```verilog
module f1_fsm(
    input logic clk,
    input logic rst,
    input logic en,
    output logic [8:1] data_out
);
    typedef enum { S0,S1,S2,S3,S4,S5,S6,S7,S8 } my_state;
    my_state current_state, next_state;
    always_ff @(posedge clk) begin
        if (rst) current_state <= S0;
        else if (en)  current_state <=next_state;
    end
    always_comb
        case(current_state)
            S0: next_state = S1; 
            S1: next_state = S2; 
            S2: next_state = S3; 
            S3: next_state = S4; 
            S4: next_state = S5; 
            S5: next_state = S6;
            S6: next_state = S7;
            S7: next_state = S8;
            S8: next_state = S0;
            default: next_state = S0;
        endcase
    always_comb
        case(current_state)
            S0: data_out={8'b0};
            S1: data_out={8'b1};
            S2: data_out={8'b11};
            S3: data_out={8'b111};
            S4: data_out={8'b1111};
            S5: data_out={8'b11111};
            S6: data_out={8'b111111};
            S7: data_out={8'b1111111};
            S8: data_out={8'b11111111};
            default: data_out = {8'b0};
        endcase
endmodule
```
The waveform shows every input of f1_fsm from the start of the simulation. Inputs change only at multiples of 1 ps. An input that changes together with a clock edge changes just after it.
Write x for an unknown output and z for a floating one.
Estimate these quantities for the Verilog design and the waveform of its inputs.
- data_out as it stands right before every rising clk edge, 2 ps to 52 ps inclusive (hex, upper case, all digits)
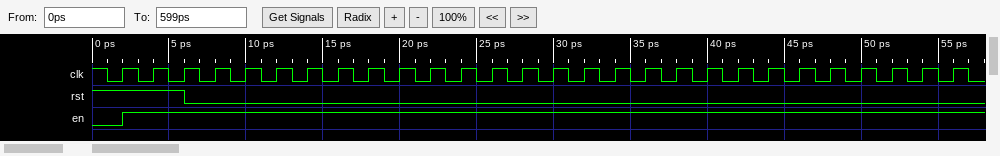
00, 00, 00, 00, 01, 03, 07, 0F, 1F, 3F, 7F, FF, 00, 01, 03, 07, 0F, 1F, 3F, 7F, FF, 00, 01, 03, 07, 0F
